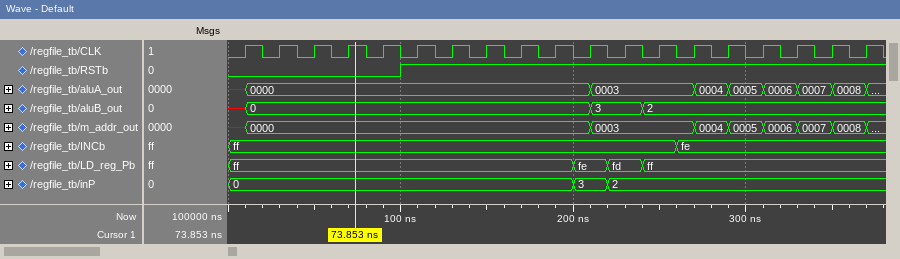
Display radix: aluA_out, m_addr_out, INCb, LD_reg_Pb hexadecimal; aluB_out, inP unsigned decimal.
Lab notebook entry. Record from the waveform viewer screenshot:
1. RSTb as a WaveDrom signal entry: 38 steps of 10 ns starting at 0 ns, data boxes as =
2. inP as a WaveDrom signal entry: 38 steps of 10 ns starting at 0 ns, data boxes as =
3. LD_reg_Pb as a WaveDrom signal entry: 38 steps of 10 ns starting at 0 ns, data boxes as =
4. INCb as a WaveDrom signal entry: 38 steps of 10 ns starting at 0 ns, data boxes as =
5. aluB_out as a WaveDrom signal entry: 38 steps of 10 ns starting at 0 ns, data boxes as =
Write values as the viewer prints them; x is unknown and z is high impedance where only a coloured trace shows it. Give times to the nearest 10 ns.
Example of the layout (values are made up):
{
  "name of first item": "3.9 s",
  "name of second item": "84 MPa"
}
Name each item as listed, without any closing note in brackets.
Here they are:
{
  "RSTb as a WaveDrom signal entry: 38 steps of 10 ns starting at 0 ns, data boxes as =": "{name: 'RSTb', wave: '0.........1...........................'}",
  "inP as a WaveDrom signal entry: 38 steps of 10 ns starting at 0 ns, data boxes as =": "{name: 'inP', wave: '=...................=.=...............', data: '0 3 2'}",
  "LD_reg_Pb as a WaveDrom signal entry: 38 steps of 10 ns starting at 0 ns, data boxes as =": "{name: 'LD_reg_Pb', wave: '=...................=.=.=.............', data: 'ff fe fd ff'}",
  "INCb as a WaveDrom signal entry: 38 steps of 10 ns starting at 0 ns, data boxes as =": "{name: 'INCb', wave: '=.........................=...........', data: 'ff fe'}",
  "aluB_out as a WaveDrom signal entry: 38 steps of 10 ns starting at 0 ns, data boxes as =": "{name: 'aluB_out', wave: 'x=...................=..=.............', data: '0 3 2'}"
}
